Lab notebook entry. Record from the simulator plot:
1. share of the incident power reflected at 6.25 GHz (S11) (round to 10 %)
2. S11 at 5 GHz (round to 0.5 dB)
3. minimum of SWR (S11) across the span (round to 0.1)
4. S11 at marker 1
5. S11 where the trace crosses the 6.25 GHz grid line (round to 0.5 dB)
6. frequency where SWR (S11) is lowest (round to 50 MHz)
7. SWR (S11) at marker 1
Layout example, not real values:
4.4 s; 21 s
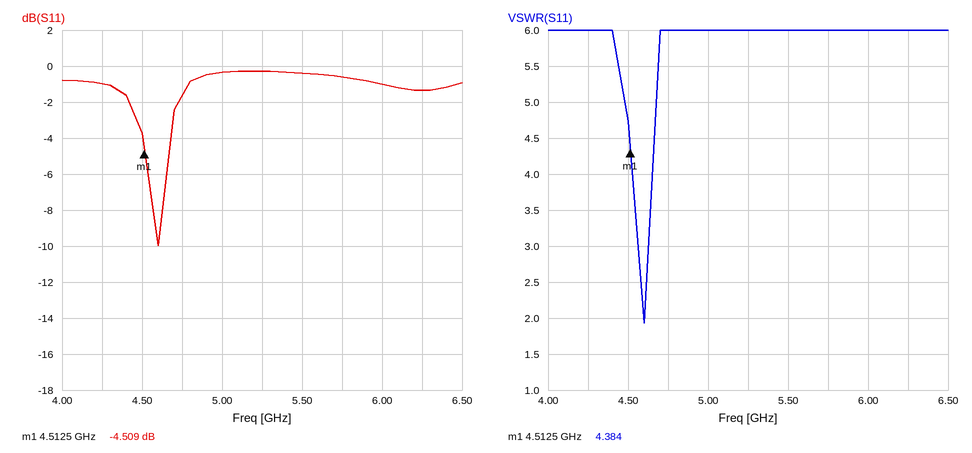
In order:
70 %; -0.5 dB; 1.9; -4.509 dB; -1.5 dB; 4.60 GHz; 4.384
